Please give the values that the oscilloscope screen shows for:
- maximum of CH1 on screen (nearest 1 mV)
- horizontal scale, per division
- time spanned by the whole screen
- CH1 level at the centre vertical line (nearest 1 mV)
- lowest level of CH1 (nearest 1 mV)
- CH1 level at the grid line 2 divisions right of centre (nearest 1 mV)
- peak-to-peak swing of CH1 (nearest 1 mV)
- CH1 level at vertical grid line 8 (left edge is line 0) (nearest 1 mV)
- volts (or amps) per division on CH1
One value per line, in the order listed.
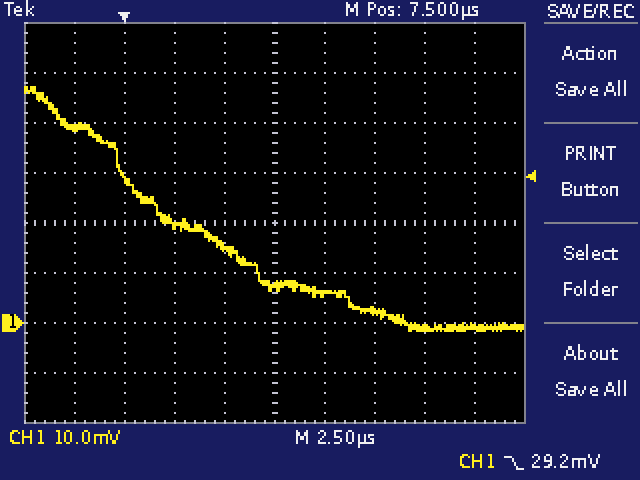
47 mV
2.5 µs
25 µs
7 mV
-2 mV
2 mV
49 mV
-1 mV
10 mV
